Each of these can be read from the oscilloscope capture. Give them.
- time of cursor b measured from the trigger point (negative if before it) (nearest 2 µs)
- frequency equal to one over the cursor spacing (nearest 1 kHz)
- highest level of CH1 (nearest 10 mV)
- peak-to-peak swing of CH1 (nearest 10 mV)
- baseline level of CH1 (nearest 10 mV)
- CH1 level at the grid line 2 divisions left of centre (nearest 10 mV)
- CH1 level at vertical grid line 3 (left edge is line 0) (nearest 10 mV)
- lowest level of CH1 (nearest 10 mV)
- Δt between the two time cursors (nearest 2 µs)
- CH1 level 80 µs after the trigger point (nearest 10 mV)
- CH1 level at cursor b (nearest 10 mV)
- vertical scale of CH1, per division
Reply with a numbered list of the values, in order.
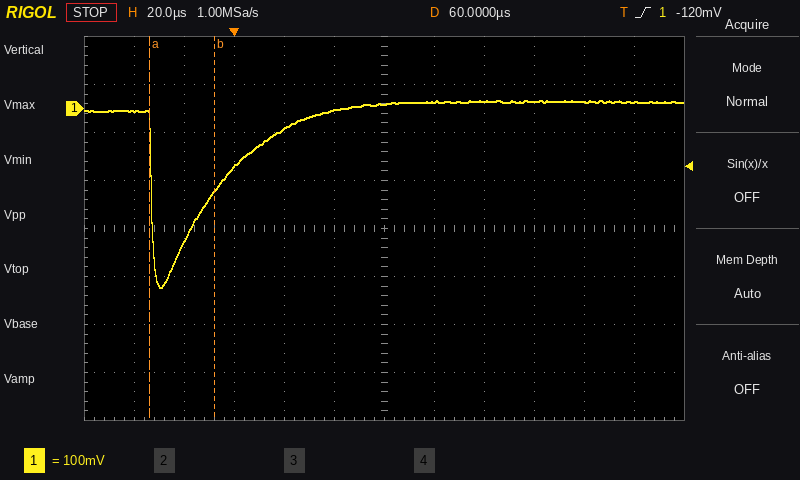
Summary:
1. -8 µs
2. 38 kHz
3. 20 mV
4. 390 mV
5. 10 mV
6. -40 mV
7. -120 mV
8. -370 mV
9. 26 µs
10. 10 mV
11. -170 mV
12. 100 mV
